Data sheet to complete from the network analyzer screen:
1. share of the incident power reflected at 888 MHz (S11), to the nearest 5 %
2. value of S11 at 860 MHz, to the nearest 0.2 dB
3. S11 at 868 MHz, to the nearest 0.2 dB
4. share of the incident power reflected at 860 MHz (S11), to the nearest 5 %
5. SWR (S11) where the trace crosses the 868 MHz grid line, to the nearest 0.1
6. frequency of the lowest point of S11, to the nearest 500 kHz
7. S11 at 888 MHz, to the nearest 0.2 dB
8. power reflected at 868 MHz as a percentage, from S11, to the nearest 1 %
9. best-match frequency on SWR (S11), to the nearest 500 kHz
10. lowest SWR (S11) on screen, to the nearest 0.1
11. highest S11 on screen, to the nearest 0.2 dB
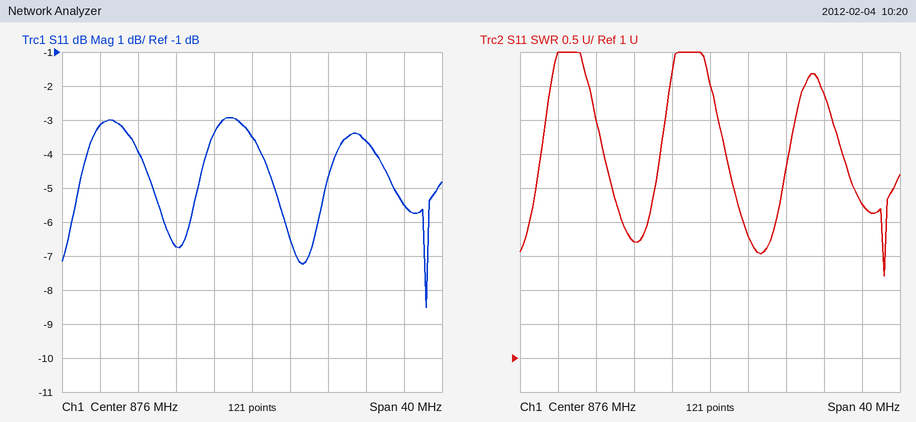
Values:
45 %
-3.2 dB
-6.8 dB
50 %
2.7
894.5 MHz
-3.6 dB
21 %
894.5 MHz
2.2
-3.0 dB
